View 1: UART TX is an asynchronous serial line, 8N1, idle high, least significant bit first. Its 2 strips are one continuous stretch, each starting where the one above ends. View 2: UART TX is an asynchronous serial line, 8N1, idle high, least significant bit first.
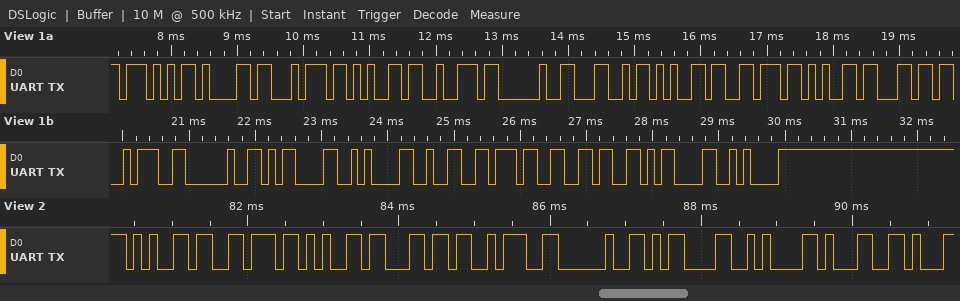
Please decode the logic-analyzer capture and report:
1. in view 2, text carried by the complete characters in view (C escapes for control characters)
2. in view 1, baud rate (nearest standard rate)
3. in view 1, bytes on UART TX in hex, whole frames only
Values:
"evel: \r\n1"
9600 baud
0x57 0x61 0x74 0x65 0x72 0x20 0x4C 0x65 0x76 0x65 0x6C 0x3A 0x20 0x0D 0x0A 0x32 0x37 0x36 0x0D 0x0A
